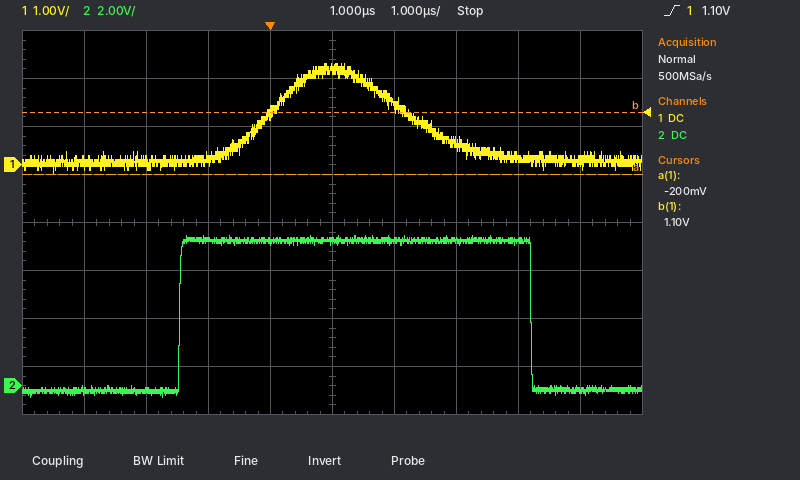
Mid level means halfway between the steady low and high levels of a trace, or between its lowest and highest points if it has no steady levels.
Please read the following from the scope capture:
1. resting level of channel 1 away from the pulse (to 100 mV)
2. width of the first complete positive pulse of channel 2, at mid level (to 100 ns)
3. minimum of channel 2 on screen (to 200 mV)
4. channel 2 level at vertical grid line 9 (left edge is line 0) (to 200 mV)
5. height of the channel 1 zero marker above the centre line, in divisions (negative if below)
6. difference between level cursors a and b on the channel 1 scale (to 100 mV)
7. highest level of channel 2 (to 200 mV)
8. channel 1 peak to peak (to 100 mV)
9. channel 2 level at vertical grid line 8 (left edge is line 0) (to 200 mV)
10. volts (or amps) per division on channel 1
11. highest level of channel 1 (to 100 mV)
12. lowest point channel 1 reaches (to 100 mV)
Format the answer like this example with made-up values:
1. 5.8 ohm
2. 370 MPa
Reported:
1. 100 mV
2. 5.7 µs
3. -400 mV
4. -200 mV
5. +1.2 div
6. 1.3 V
7. 6.2 V
8. 2.3 V
9. 6.0 V
10. 1 V
11. 2.1 V
12. -200 mV
